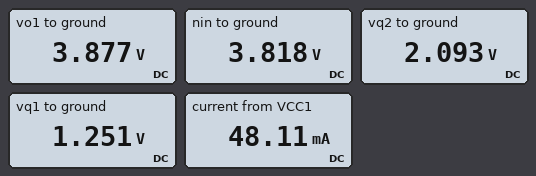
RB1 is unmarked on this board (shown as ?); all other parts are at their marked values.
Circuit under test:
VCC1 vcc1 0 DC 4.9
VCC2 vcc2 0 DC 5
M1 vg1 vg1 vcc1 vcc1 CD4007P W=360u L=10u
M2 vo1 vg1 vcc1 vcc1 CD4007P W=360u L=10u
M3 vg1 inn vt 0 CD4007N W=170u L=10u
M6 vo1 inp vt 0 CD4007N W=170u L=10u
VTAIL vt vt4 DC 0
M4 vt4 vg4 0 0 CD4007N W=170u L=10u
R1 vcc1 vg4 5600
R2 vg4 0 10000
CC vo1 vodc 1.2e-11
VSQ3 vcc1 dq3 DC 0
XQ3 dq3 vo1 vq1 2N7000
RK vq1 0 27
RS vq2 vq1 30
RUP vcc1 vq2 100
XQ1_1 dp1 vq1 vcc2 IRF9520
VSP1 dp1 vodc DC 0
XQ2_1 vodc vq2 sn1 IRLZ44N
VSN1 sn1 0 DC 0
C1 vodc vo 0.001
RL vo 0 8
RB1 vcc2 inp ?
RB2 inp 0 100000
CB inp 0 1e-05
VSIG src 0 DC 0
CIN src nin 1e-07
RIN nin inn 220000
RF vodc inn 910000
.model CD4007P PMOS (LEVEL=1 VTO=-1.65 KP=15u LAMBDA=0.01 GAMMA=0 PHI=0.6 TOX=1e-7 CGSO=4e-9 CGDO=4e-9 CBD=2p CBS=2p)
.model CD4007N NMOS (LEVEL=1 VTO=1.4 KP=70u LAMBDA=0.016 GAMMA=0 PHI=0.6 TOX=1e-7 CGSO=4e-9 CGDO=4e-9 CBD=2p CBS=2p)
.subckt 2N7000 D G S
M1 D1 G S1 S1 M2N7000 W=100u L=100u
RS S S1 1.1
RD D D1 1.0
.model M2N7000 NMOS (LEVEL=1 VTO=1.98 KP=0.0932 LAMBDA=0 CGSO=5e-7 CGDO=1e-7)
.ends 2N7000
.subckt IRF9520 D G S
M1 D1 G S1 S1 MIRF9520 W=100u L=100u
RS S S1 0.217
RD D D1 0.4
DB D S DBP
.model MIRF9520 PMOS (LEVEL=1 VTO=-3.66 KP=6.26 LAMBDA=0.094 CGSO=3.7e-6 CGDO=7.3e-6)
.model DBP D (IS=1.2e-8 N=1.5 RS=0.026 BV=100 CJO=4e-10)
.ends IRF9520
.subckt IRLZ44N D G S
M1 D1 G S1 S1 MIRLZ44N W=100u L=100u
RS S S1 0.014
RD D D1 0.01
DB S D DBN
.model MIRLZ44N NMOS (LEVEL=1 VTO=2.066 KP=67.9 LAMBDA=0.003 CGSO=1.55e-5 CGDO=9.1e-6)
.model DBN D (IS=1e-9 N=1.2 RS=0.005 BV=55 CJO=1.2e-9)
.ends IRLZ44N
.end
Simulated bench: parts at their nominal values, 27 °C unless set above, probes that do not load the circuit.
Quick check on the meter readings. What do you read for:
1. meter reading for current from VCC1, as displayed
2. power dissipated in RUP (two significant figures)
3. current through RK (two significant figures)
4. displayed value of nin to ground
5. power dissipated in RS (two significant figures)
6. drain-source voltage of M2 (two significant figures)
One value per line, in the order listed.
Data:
48.11 mA
79 mW
46 mA
3.818 V
24 mW
-1.0 V
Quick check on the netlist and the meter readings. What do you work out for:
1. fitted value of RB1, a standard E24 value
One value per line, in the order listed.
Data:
47 kΩ
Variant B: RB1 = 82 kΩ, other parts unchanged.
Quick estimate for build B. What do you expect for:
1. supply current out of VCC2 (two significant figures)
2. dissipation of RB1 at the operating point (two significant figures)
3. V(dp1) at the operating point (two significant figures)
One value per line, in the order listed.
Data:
26 mA
62 µW
2.8 V
